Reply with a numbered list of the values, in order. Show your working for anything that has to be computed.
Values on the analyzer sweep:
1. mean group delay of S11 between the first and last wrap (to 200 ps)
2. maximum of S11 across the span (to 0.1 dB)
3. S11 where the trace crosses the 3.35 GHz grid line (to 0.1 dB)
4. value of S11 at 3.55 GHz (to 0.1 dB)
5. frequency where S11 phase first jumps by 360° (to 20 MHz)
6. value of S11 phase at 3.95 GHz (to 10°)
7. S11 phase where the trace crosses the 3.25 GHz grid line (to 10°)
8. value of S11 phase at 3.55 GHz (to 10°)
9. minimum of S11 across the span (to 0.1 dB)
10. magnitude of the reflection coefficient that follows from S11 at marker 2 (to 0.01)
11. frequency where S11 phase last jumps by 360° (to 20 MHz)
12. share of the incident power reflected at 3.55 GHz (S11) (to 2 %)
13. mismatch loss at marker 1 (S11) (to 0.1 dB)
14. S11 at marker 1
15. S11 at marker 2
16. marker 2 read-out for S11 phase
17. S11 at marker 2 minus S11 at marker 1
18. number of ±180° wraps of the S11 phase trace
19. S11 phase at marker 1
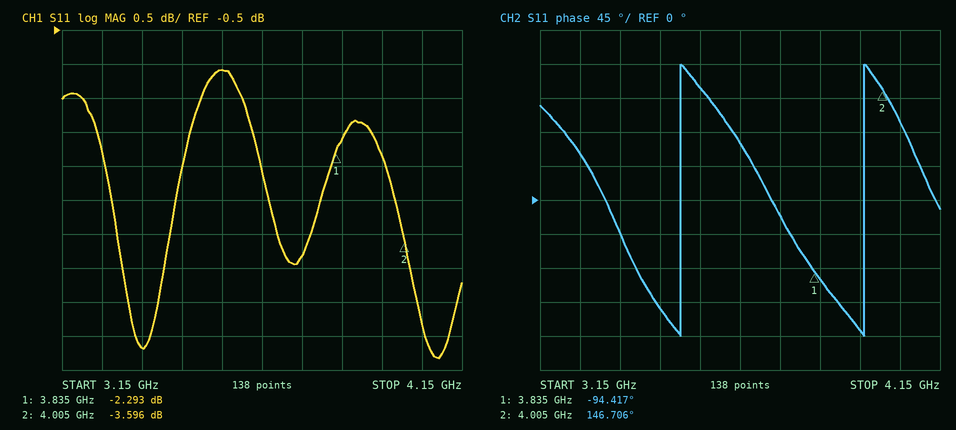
1. 1 cycle / (3.96 GHz − 3.50 GHz) ≈ 2.2 ns
2. -1.1 dB
3. -5.2 dB
4. -1.1 dB
5. 3.50 GHz
6. -170°
7. 60°
8. 150°
9. -5.3 dB
10. 10^(-3.596/20) ≈ 0.66
11. 3.96 GHz
12. 10^(-1.1/10) ≈ 78 %
13. −10 log10(1 − 10^(-2.293/10)) ≈ 3.9 dB
14. -2.293 dB
15. -3.596 dB
16. 146.706°
17. -3.596 − (-2.293) = -1.303 dB
18. 2
19. -94.417°
